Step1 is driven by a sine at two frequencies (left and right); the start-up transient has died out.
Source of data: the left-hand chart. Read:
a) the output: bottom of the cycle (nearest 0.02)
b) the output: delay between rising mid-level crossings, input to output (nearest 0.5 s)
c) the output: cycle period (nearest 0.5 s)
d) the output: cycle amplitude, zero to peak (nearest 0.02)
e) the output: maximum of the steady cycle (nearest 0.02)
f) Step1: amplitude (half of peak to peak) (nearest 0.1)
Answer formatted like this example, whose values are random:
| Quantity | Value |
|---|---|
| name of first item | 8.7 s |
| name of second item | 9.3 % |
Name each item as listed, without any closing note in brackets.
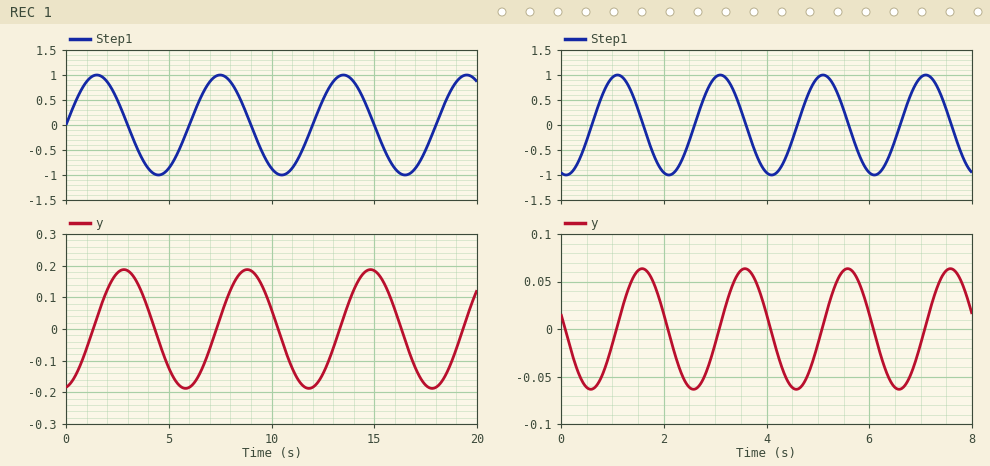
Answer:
| Quantity | Value |
|---|---|
| the output: bottom of the cycle | -0.18 |
| the output: delay between rising mid-level crossings, input to output | 1.5 s |
| the output: cycle period | 6.0 s |
| the output: cycle amplitude, zero to peak | 0.18 |
| the output: maximum of the steady cycle | 0.18 |
| Step1: amplitude (half of peak to peak) | 1.0 |
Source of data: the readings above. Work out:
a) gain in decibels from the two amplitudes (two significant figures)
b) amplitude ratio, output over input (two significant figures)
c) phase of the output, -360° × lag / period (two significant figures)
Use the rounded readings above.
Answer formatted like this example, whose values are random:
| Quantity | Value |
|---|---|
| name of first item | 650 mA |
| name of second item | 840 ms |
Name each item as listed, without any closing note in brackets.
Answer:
| Quantity | Value |
|---|---|
| gain in decibels from the two amplitudes | -15 dB |
| amplitude ratio, output over input | 0.18 |
| phase of the output, -360° × lag / period | -90° |
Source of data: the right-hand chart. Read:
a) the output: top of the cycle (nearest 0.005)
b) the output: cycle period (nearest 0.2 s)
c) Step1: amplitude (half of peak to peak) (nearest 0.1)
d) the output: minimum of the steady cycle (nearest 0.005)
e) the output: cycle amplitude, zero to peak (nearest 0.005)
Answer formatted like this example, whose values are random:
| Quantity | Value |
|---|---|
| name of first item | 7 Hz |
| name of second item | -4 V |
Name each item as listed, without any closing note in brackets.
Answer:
| Quantity | Value |
|---|---|
| the output: top of the cycle | 0.065 |
| the output: cycle period | 2.0 s |
| Step1: amplitude (half of peak to peak) | 1.0 |
| the output: minimum of the steady cycle | -0.065 |
| the output: cycle amplitude, zero to peak | 0.065 |
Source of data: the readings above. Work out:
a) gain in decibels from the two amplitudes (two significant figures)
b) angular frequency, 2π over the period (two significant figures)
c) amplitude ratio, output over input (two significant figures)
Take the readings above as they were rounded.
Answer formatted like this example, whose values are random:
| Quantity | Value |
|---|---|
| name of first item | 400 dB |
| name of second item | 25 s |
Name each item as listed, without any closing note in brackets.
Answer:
| Quantity | Value |
|---|---|
| gain in decibels from the two amplitudes | -24 dB |
| angular frequency, 2π over the period | 3.1 rad/s |
| amplitude ratio, output over input | 0.065 |
